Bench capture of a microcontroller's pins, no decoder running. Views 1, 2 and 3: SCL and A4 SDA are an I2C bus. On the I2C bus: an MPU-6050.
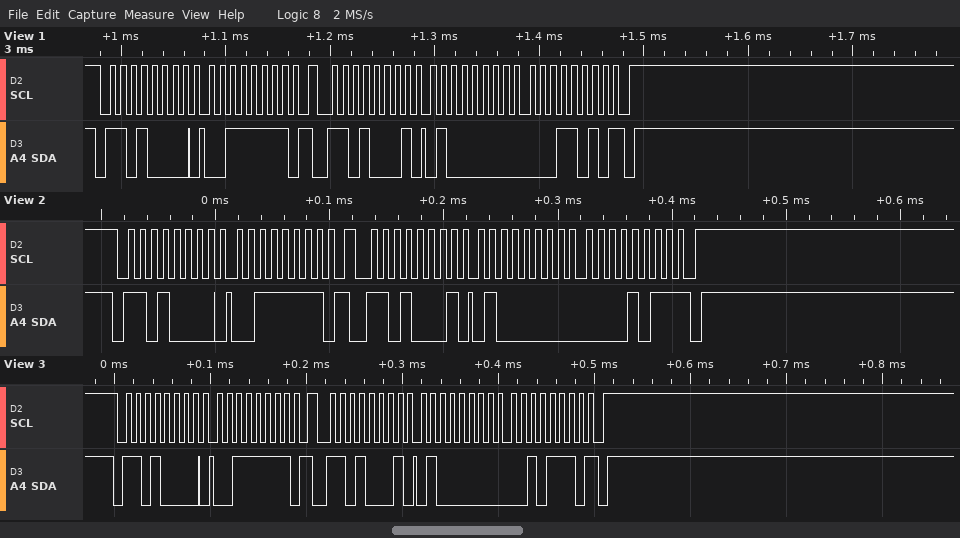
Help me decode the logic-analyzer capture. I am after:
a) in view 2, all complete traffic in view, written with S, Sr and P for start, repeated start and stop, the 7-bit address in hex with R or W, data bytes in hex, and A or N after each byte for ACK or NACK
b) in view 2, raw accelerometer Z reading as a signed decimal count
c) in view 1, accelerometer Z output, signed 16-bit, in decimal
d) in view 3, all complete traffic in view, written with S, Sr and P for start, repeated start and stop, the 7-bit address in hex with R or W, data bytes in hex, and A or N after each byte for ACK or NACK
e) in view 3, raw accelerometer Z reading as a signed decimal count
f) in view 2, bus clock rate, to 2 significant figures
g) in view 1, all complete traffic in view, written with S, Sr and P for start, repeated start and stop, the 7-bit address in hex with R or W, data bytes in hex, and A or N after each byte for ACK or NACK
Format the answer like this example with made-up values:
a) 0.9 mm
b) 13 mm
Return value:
a) S 68W A 3F A Sr 68R A 40 A 0B N P
b) 16395
c) 16410
d) S 68W A 3F A Sr 68R A 40 A 2E N P
e) 16430
f) 100 kHz
g) S 68W A 3F A Sr 68R A 40 A 1A N P
